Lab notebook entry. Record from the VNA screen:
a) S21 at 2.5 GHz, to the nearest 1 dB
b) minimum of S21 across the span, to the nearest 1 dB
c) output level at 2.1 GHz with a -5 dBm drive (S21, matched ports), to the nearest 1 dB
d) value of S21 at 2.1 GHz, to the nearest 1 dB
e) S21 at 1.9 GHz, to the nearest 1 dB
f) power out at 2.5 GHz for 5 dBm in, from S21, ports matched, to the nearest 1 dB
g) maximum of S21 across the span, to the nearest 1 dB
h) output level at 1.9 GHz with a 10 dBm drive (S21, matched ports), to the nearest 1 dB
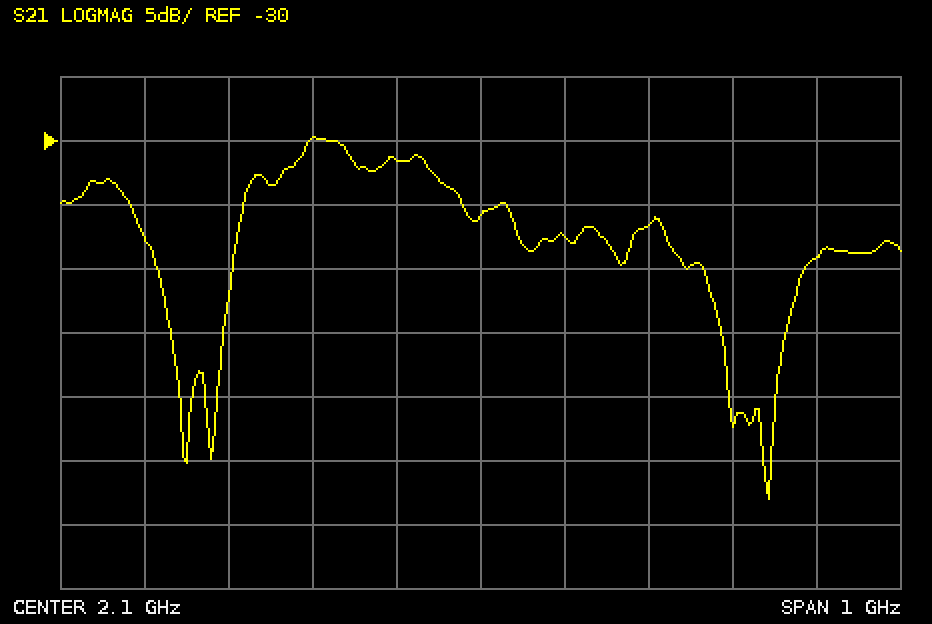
-39 dB
-58 dB
-41 dBm
-36 dB
-30 dB
-34 dBm
-30 dB
-20 dBm
